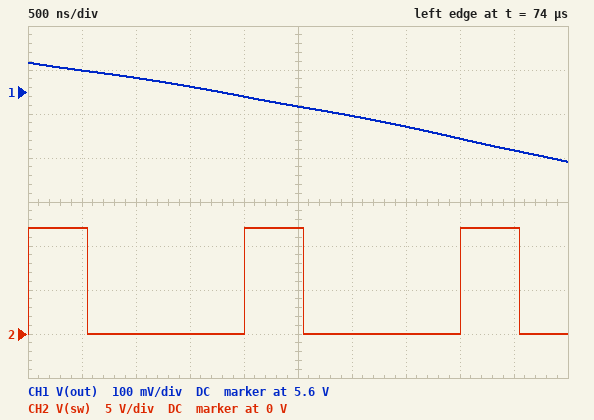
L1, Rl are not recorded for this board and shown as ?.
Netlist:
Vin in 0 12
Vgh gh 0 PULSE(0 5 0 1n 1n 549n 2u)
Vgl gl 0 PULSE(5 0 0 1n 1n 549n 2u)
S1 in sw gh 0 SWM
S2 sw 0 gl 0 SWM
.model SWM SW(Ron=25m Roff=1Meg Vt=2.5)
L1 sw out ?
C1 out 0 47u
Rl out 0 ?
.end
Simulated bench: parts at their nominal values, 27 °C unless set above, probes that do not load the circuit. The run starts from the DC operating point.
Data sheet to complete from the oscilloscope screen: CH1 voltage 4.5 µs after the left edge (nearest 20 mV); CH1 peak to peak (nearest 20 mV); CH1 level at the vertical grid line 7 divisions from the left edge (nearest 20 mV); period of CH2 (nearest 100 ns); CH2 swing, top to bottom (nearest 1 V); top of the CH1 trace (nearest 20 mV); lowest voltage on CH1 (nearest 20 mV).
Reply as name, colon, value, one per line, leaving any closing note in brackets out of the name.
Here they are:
CH1 voltage 4.5 µs after the left edge: 5.46 V
CH1 peak to peak: 220 mV
CH1 level at the vertical grid line 7 divisions from the left edge: 5.52 V
period of CH2: 2.0 µs
CH2 swing, top to bottom: 12 V
top of the CH1 trace: 5.66 V
lowest voltage on CH1: 5.44 V
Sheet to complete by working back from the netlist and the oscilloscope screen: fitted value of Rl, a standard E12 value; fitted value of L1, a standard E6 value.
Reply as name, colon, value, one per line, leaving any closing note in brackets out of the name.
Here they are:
fitted value of Rl, a standard E12 value: 3.9 Ω
fitted value of L1, a standard E6 value: 10 µH
